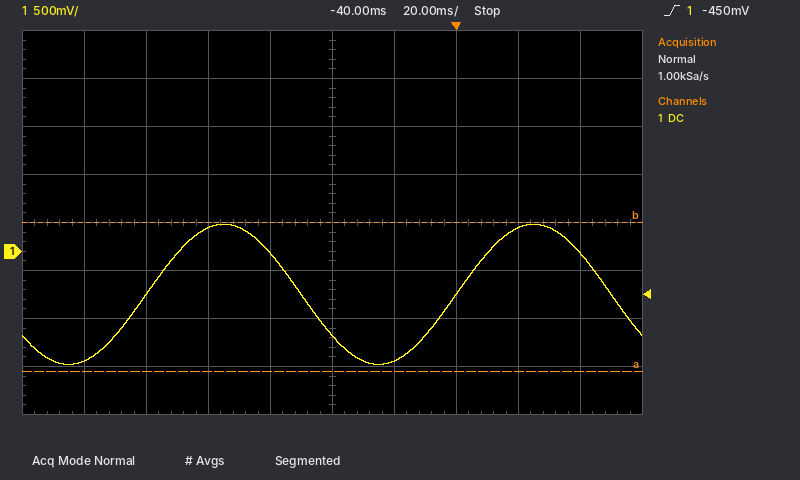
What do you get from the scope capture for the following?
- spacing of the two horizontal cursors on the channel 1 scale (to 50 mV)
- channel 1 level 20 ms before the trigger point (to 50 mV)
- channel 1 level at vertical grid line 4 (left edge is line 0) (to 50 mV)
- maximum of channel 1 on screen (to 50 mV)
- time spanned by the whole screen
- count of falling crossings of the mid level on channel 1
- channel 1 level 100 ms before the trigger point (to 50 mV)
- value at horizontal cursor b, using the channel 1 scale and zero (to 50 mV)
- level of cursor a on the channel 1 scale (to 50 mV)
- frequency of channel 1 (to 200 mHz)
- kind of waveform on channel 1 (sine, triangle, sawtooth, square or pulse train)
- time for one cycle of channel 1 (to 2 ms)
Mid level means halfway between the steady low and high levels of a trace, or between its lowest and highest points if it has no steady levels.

1.55 V
-1.15 V
0 mV
300 mV
200 ms
2
-450 mV
300 mV
-1.25 V
10.0 Hz
sine
100 ms
